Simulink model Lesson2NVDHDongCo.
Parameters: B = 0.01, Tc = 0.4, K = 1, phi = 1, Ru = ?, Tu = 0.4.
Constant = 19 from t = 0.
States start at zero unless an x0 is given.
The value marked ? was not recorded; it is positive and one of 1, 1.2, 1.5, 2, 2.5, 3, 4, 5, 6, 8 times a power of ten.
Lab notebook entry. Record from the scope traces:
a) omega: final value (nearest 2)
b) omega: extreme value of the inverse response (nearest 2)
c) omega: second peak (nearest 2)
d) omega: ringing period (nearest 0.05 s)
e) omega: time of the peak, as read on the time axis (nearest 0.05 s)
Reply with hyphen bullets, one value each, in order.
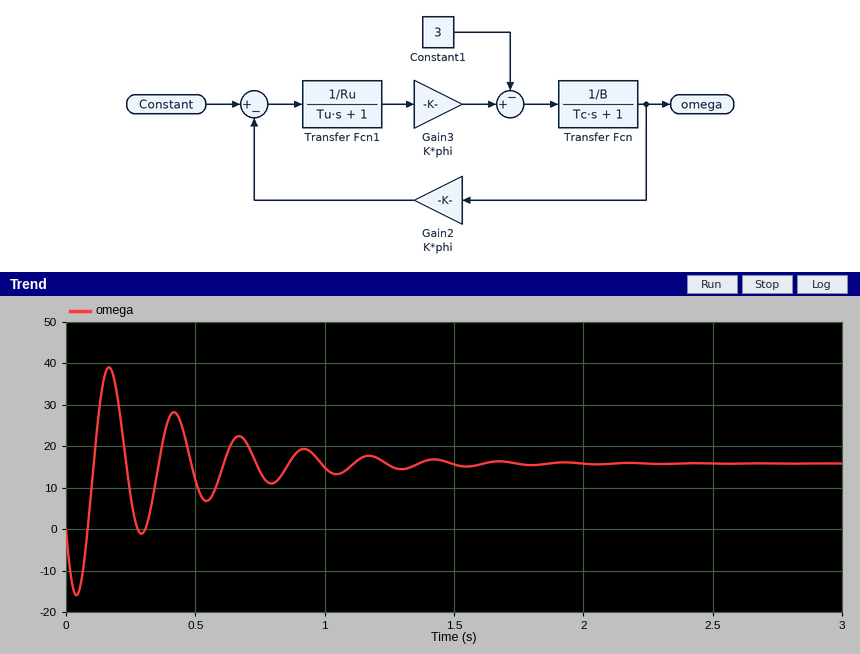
- 16
- -16
- 28
- 0.25 s
- 0.15 s
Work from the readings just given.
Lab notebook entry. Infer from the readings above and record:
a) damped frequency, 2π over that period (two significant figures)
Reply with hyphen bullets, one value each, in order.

- 25 rad/s
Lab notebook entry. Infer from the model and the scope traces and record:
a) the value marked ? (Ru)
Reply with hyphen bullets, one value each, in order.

- 1
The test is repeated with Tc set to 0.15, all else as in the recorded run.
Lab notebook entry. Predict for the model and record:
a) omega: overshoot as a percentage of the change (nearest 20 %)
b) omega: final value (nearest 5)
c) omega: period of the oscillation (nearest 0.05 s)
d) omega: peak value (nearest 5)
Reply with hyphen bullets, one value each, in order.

- 200 %
- 15
- 0.15 s
- 50
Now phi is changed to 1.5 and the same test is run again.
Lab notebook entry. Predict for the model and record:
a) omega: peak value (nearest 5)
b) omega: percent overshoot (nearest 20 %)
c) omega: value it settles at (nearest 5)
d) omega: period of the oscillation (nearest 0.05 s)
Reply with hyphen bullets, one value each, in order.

- 30
- 160 %
- 10
- 0.15 s
